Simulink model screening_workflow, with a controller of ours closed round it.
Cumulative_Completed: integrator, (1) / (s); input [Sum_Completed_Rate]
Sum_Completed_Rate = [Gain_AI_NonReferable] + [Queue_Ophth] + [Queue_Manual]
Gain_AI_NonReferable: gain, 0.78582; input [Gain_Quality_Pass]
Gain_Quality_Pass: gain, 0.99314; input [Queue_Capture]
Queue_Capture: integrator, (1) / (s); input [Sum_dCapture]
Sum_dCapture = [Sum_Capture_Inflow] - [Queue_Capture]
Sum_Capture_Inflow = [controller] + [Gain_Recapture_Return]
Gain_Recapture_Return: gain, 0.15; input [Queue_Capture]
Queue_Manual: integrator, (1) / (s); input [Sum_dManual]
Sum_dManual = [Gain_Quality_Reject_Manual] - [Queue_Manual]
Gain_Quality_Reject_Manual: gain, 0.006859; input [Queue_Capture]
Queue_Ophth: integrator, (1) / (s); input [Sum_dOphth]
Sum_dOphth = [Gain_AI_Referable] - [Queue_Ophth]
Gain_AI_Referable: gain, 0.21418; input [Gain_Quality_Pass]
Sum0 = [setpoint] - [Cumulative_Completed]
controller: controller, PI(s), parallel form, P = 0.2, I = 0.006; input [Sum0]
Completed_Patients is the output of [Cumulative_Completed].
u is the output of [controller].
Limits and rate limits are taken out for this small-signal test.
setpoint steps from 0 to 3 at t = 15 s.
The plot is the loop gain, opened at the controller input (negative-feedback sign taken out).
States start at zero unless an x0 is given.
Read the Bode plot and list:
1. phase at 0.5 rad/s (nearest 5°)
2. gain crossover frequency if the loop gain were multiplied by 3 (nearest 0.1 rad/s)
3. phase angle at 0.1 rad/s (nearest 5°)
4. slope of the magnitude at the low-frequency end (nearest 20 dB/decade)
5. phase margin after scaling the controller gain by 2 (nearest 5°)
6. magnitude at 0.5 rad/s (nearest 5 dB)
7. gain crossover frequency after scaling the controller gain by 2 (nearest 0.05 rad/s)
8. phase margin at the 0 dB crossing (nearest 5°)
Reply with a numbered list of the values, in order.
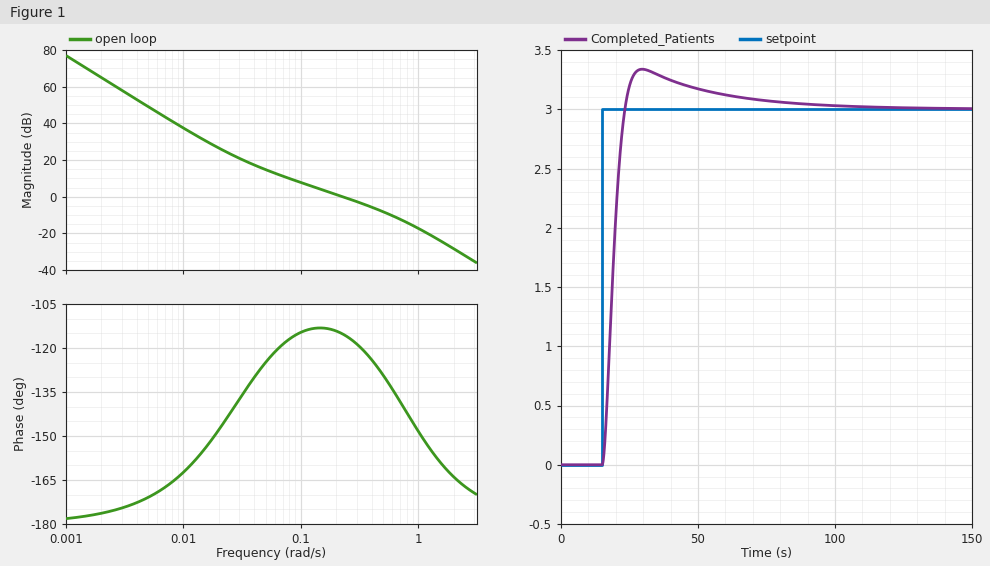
1. -130°
2. 0.6 rad/s
3. -115°
4. -40 dB/decade
5. 55°
6. -10 dB
7. 0.40 rad/s
8. 65°
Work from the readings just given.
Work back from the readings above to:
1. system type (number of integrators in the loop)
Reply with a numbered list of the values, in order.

1. 2
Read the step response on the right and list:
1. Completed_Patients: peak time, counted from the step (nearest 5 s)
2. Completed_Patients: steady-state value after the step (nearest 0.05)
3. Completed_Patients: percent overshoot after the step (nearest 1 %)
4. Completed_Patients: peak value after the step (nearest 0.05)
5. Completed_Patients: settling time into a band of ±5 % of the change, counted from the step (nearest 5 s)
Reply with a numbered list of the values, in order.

1. 15 s
2. 3.00
3. 11 %
4. 3.35
5. 40 s
